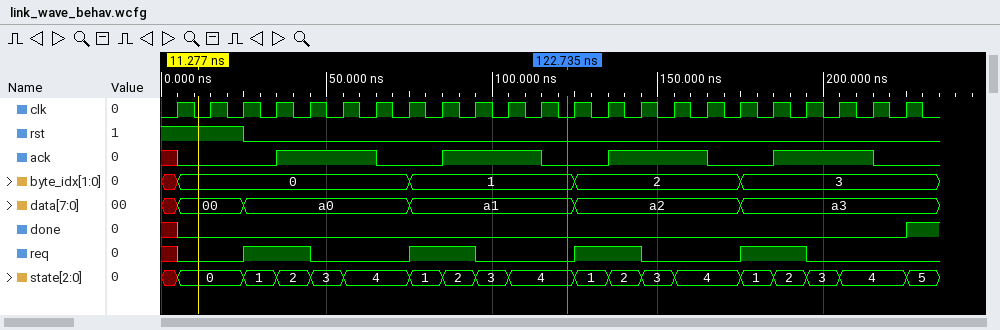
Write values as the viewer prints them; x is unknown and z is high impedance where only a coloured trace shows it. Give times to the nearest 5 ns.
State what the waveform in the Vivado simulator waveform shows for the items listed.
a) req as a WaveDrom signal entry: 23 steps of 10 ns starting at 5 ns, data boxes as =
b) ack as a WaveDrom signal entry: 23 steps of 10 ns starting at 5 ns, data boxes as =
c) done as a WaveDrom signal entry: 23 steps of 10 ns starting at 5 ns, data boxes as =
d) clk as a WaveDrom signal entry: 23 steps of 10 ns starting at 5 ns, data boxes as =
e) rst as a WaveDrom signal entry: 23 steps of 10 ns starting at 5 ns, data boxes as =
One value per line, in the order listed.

{name: 'req', wave: '0.1.0..1.0..1.0..1.0...'}
{name: 'ack', wave: '0..1..0.1..0.1..0.1..0.'}
{name: 'done', wave: '0.....................1'}
{name: 'clk', wave: 'p......................'}
{name: 'rst', wave: '1.0....................'}
